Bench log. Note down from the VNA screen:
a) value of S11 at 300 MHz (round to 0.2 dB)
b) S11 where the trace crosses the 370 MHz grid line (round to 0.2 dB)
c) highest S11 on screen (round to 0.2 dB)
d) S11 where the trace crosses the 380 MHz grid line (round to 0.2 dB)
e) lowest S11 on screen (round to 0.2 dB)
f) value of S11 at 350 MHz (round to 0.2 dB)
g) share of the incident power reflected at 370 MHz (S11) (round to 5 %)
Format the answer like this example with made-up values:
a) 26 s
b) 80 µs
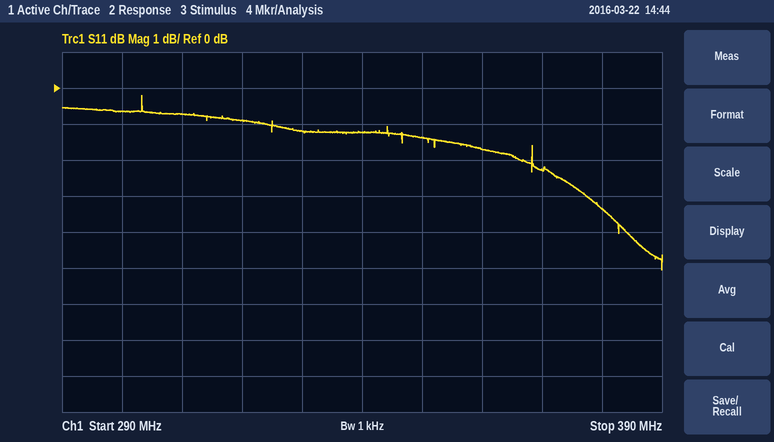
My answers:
a) -0.6 dB
b) -2.2 dB
c) -0.2 dB
d) -3.4 dB
e) -5.0 dB
f) -1.4 dB
g) 60 %
